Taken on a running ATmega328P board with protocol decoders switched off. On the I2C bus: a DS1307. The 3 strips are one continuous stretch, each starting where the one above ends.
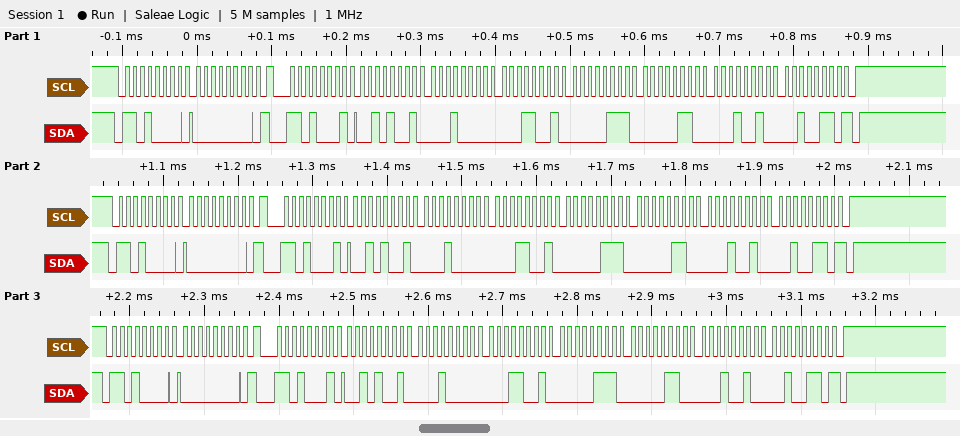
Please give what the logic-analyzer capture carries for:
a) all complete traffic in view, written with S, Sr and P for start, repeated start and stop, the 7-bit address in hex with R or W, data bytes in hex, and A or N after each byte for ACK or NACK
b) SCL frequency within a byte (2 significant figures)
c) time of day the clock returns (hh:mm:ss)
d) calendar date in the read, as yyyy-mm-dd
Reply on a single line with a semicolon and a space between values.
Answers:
S 68W A 00 A Sr 68R A 29 A 10 A 19 A 07 A 06 A 12 A 26 N P S 68W A 00 A Sr 68R A 29 A 10 A 19 A 07 A 06 A 12 A 26 N P S 68W A 00 A Sr 68R A 29 A 10 A 19 A 07 A 06 A 12 A 26 N P; 100 kHz; 19:10:29; 2026-12-06
